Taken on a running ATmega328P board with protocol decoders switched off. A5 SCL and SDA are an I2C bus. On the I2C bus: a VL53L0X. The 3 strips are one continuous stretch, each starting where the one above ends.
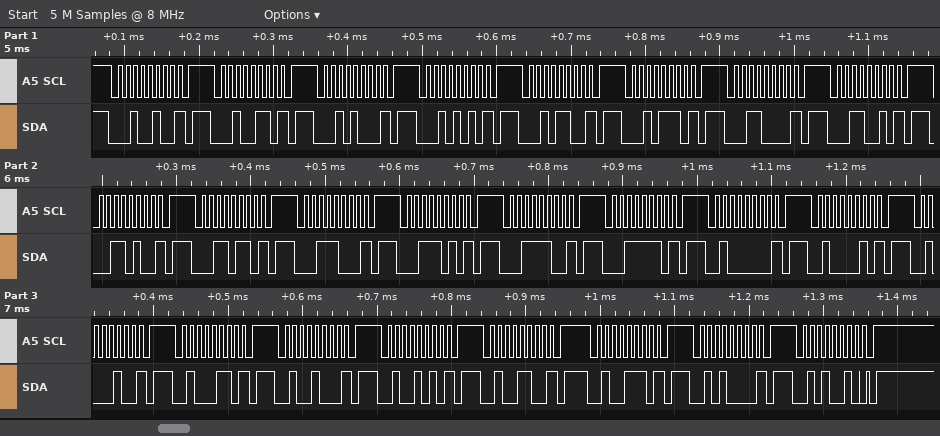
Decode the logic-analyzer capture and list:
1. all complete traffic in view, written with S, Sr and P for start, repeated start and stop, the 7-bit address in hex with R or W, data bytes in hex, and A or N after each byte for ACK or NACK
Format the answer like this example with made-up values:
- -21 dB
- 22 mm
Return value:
- S 12W N P S 13W N P S 14W N P S 15W N P S 16W N P S 17W N P S 18W N P S 19W N P S 1AW N P S 1BW N P S 1CW N P S 1DW N P S 1EW N P S 1FW N P S 20W N P S 21W N P S 22W N P S 23W N P S 24W N P S 25W N P S 26W N P S 27W N P S 28W N P S 29W A P
